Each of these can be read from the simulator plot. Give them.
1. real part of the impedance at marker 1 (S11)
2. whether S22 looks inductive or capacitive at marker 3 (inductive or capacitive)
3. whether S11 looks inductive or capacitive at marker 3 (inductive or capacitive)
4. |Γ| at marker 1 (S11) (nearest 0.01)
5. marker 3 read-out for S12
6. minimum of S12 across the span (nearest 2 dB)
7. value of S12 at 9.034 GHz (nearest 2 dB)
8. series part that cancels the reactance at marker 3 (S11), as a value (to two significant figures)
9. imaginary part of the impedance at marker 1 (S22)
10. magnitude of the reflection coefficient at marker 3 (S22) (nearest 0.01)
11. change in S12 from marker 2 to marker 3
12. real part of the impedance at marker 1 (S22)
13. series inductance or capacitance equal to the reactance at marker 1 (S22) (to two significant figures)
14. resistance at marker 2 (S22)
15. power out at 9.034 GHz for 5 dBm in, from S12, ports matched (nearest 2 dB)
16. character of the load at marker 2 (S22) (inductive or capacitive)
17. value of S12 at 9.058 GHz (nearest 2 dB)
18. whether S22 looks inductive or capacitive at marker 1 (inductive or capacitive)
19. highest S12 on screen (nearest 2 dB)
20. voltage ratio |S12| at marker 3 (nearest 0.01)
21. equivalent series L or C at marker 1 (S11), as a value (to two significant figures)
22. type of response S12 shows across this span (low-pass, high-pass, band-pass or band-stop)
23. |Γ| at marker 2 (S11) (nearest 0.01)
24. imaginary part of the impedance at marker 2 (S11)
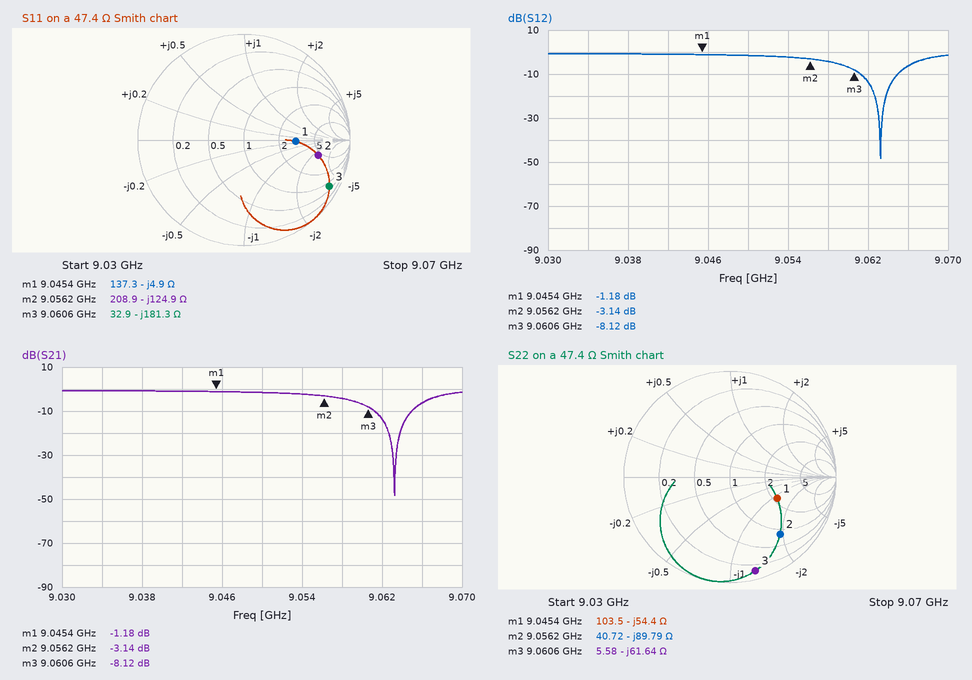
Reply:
137.3 Ω
capacitive
capacitive
0.49
-8.12 dB
-48 dB
0 dB
3.2 nH
-54.4 Ω
0.92
-4.98 dB
103.5 Ω
320 fF
40.72 Ω
4 dBm
capacitive
-4 dB
capacitive
0 dB
0.39
3.6 pF
band-stop
0.72
-124.9 Ω
